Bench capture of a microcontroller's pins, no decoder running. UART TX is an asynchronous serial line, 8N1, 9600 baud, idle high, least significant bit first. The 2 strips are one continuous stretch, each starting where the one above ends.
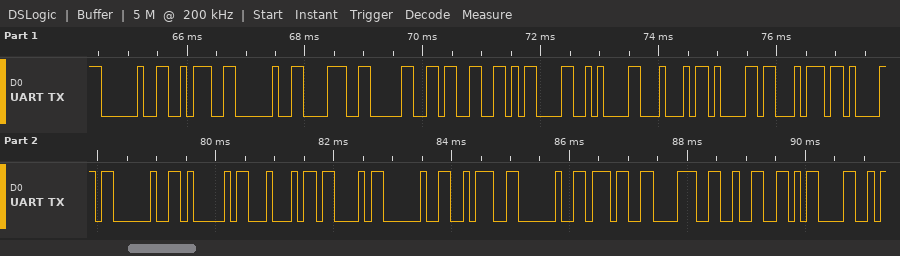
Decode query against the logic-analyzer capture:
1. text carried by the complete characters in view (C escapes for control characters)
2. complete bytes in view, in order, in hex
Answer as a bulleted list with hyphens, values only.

- " : 803\r\nData ADC : 782\r"
- 20 3A 20 38 30 33 0D 0A 44 61 74 61 20 41 44 43 20 3A 20 37 38 32 0D
